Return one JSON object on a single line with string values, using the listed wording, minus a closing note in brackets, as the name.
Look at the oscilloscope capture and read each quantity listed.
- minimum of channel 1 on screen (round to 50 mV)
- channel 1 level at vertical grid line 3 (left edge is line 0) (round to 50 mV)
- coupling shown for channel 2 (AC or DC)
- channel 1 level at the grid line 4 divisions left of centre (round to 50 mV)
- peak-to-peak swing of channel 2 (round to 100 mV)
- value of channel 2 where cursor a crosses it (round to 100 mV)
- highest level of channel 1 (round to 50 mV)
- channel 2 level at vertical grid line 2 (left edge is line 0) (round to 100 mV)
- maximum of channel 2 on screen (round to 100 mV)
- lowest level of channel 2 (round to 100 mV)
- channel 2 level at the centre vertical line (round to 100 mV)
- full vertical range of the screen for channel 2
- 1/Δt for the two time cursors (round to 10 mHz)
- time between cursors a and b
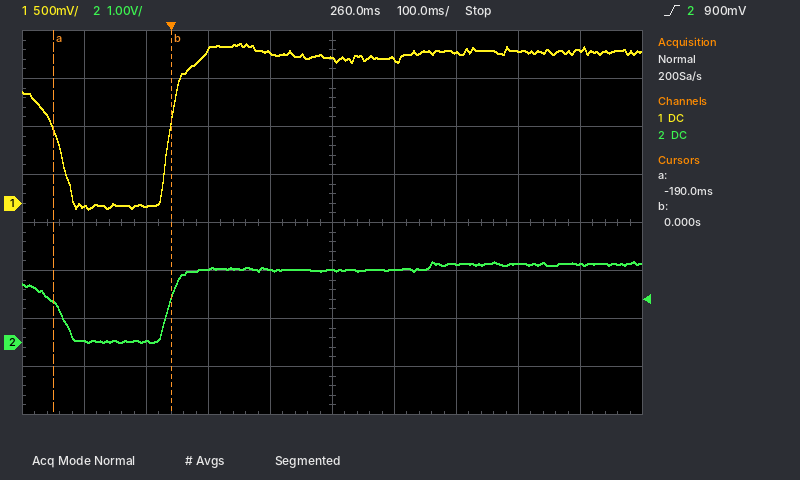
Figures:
{"minimum of channel 1 on screen": "-50 mV", "channel 1 level at vertical grid line 3 (left edge is line 0)": "1.60 V", "coupling shown for channel 2": "DC", "channel 1 level at the grid line 4 divisions left of centre": "-50 mV", "peak-to-peak swing of channel 2": "1.7 V", "value of channel 2 where cursor a crosses it": "800 mV", "highest level of channel 1": "1.65 V", "channel 2 level at vertical grid line 2 (left edge is line 0)": "0.0 V", "maximum of channel 2 on screen": "1.7 V", "lowest level of channel 2": "0.0 V", "channel 2 level at the centre vertical line": "1.5 V", "full vertical range of the screen for channel 2": "8 V", "1/Δt for the two time cursors": "5.26 Hz", "time between cursors a and b": "190 ms"}
